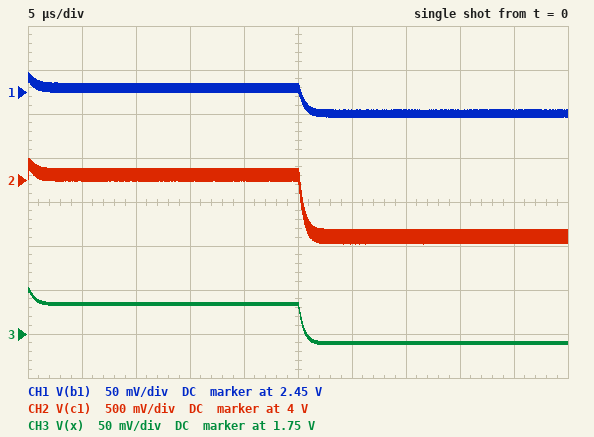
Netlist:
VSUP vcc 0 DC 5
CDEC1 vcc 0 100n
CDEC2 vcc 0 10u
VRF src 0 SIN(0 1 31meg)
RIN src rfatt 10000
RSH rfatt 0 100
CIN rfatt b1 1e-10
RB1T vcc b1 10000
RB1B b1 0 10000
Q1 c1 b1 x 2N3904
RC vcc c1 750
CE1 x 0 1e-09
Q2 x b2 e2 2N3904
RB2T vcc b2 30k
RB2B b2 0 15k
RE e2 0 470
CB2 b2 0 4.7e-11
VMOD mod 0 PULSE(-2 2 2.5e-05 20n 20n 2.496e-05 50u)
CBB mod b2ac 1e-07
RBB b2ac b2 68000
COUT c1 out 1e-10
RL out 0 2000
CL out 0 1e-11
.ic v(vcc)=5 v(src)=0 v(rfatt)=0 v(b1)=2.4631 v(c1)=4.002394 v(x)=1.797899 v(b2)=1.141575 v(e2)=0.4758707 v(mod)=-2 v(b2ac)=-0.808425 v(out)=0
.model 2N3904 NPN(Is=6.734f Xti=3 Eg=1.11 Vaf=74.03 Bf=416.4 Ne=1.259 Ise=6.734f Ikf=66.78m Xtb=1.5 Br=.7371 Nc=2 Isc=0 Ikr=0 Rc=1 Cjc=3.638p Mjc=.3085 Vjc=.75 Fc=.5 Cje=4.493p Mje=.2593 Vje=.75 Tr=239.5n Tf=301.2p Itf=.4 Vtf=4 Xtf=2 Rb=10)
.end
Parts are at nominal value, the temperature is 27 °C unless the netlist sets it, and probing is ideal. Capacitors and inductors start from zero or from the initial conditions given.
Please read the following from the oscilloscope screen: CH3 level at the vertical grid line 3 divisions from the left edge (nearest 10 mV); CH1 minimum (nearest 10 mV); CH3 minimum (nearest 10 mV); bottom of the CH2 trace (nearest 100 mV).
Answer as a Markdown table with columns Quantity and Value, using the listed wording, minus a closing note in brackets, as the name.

| Quantity | Value |
|---|---|
| CH3 level at the vertical grid line 3 divisions from the left edge | 1.78 V |
| CH1 minimum | 2.42 V |
| CH3 minimum | 1.74 V |
| bottom of the CH2 trace | 3.3 V |
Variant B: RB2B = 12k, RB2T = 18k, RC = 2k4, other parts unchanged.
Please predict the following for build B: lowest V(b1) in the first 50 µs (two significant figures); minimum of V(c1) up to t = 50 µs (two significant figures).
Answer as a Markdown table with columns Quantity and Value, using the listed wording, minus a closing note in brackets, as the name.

| Quantity | Value |
|---|---|
| lowest V(b1) in the first 50 µs | 1.7 V |
| minimum of V(c1) up to t = 50 µs | 1.1 V |
